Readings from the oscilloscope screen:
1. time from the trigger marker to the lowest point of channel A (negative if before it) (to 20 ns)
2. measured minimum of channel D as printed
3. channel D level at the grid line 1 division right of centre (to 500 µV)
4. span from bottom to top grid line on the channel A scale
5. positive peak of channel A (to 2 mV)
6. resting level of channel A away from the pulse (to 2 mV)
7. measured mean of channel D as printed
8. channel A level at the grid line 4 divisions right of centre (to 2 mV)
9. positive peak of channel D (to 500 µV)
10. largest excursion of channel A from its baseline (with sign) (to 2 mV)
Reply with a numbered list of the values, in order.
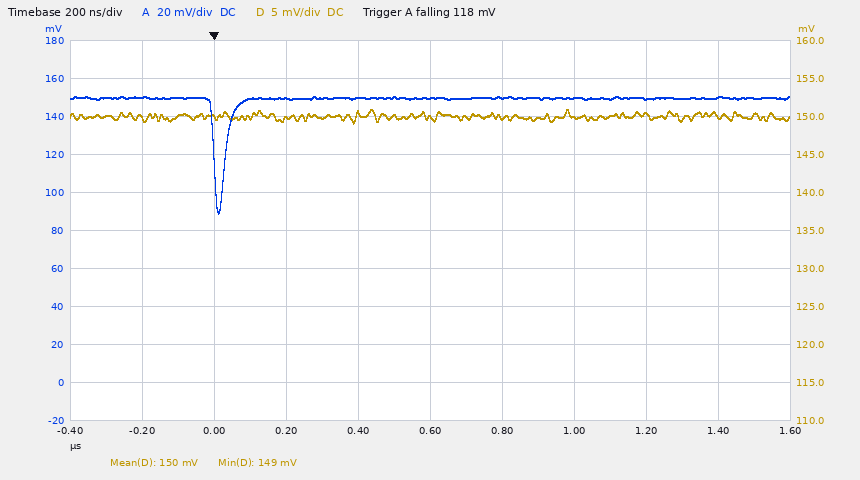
1. +20 ns
2. 149 mV
3. 150.0 mV
4. 200 mV
5. 150 mV
6. 150 mV
7. 150 mV
8. 150 mV
9. 151.0 mV
10. -60 mV
